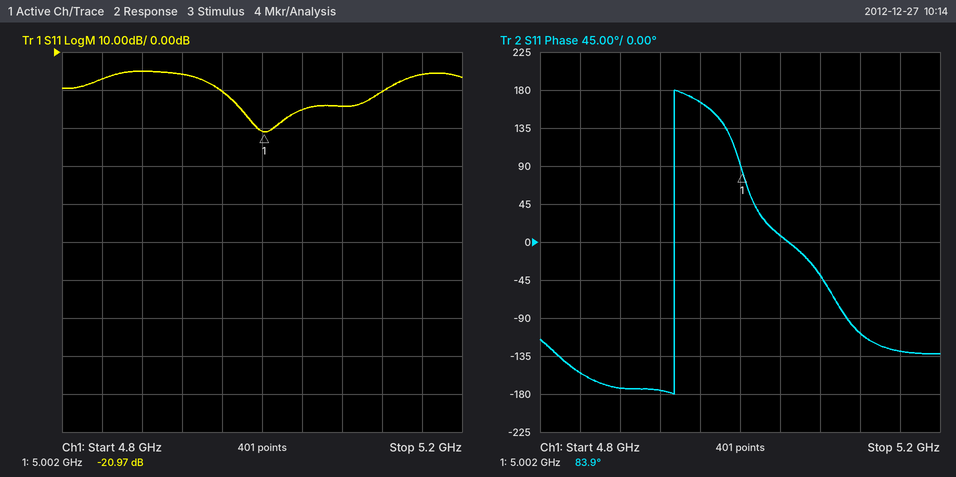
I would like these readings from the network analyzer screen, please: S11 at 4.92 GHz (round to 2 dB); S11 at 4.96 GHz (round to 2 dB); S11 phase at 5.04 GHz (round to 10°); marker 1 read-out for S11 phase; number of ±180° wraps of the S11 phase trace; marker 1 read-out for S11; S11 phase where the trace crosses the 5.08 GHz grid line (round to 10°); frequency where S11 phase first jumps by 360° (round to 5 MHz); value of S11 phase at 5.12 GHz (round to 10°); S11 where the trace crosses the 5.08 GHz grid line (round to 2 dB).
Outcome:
-6 dB
-10 dB
10°
83.9°
1
-20.97 dB
-40°
4.935 GHz
-110°
-14 dB
